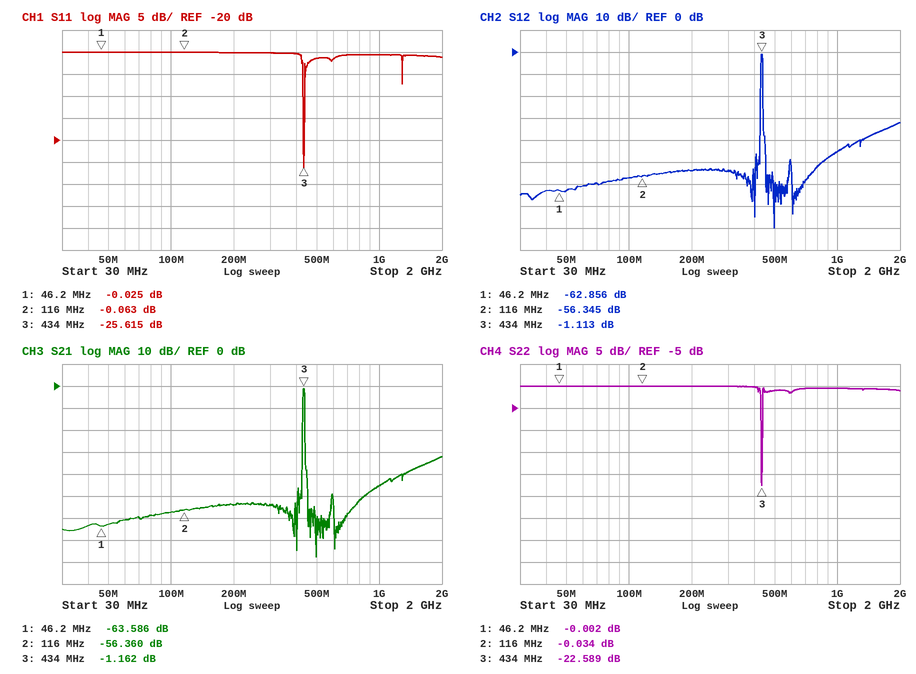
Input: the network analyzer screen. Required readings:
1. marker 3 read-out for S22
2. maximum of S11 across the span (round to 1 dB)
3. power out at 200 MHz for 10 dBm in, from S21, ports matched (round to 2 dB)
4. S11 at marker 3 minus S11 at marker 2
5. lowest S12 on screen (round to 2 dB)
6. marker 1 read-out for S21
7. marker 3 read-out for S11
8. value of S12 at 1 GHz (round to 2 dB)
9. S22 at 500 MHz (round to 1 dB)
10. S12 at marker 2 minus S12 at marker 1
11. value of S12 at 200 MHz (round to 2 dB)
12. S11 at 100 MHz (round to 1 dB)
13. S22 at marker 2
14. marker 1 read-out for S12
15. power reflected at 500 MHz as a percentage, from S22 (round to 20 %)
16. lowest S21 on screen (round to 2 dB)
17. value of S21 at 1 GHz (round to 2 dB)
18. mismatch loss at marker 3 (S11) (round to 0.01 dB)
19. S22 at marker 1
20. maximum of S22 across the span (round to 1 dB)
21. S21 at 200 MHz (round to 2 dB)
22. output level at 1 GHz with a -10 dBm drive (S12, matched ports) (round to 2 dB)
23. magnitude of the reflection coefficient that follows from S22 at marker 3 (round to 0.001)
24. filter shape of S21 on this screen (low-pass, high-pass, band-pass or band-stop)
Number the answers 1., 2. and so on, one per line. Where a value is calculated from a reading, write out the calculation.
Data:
1. -22.589 dB
2. 0 dB
3. 10 dBm + (-54 dB) = -44 dBm
4. -25.615 − (-0.063) = -25.552 dB
5. -80 dB
6. -63.586 dB
7. -25.615 dB
8. -46 dB
9. -1 dB
10. -56.345 − (-62.856) = 6.511 dB
11. -54 dB
12. 0 dB
13. -0.034 dB
14. -62.856 dB
15. 10^(-1/10) ≈ 79.4 %, so 80 % to the nearest 20 %
16. -78 dB
17. -46 dB
18. −10 log10(1 − 10^(-25.615/10)) ≈ 0.01 dB
19. -0.002 dB
20. 0 dB
21. -54 dB
22. -10 dBm + (-46 dB) = -56 dBm
23. 10^(-22.589/20) ≈ 0.074
24. band-pass
